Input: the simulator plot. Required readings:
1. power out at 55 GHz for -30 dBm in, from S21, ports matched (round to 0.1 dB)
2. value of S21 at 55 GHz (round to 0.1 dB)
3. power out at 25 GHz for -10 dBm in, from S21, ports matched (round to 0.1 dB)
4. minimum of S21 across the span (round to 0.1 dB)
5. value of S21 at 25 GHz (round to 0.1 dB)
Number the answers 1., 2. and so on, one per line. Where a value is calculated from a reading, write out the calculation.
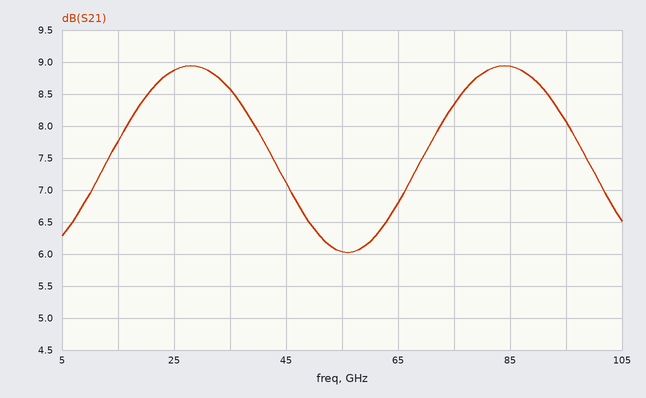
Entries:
1. -30 dBm + (6.0 dB) = -24.0 dBm
2. 6.0 dB
3. -10 dBm + (8.9 dB) = -1.1 dBm
4. 6.0 dB
5. 8.9 dB
